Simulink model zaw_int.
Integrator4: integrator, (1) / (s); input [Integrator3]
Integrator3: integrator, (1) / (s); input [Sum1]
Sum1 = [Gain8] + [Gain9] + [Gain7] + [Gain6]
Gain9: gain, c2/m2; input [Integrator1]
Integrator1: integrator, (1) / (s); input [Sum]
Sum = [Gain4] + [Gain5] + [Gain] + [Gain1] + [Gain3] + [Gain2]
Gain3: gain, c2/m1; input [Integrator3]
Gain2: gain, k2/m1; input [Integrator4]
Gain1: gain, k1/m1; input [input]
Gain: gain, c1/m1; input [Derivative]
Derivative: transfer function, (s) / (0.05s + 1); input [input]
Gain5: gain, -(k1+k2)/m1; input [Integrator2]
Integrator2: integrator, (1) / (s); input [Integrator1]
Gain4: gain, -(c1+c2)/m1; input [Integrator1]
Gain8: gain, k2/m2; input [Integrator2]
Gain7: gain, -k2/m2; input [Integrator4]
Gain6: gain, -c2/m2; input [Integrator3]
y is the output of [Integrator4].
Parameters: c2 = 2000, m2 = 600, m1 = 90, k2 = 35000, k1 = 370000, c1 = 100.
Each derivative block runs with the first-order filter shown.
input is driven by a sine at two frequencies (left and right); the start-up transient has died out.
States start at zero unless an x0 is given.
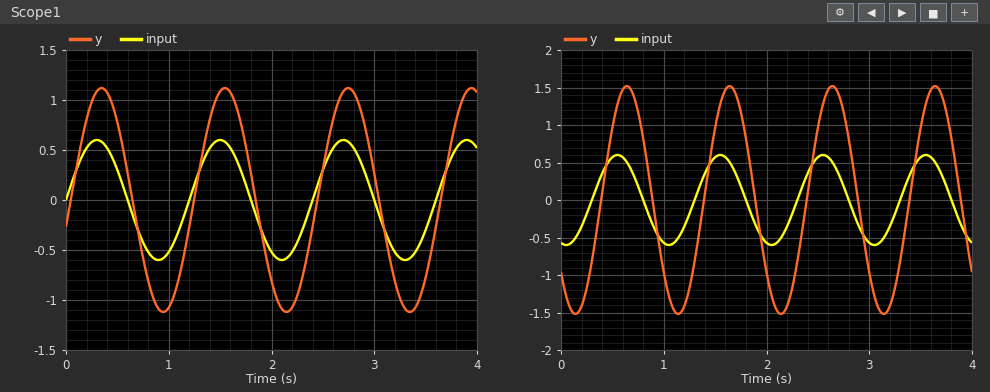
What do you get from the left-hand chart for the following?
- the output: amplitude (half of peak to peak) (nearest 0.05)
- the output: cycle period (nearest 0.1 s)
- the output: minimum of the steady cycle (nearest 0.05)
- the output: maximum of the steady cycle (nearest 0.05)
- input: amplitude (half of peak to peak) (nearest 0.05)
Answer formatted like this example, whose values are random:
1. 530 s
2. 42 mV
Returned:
1. 1.10
2. 1.2 s
3. -1.10
4. 1.10
5. 0.60
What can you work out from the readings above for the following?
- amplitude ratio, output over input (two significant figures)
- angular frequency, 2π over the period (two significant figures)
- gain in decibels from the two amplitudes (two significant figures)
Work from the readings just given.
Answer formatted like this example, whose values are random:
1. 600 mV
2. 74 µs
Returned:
1. 1.8
2. 5.2 rad/s
3. 5.3 dB
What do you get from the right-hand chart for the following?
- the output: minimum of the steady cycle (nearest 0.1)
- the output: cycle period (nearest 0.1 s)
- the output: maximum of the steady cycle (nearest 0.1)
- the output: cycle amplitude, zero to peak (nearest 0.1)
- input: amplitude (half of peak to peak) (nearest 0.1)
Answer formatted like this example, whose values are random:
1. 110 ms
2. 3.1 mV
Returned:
1. -1.5
2. 1.0 s
3. 1.5
4. 1.5
5. 0.6
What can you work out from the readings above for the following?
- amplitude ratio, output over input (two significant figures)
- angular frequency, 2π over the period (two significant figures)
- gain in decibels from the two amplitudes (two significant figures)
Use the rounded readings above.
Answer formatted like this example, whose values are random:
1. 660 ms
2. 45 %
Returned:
1. 2.5
2. 6.3 rad/s
3. 8.0 dB
